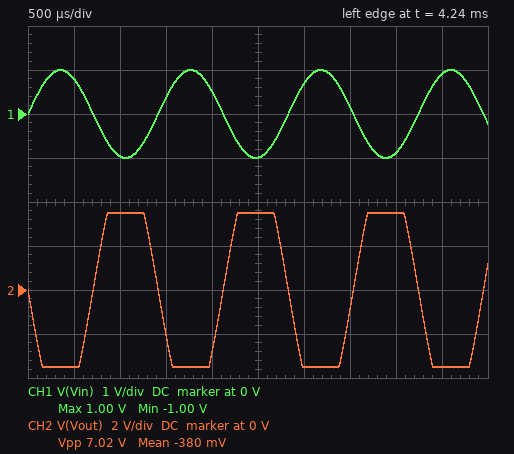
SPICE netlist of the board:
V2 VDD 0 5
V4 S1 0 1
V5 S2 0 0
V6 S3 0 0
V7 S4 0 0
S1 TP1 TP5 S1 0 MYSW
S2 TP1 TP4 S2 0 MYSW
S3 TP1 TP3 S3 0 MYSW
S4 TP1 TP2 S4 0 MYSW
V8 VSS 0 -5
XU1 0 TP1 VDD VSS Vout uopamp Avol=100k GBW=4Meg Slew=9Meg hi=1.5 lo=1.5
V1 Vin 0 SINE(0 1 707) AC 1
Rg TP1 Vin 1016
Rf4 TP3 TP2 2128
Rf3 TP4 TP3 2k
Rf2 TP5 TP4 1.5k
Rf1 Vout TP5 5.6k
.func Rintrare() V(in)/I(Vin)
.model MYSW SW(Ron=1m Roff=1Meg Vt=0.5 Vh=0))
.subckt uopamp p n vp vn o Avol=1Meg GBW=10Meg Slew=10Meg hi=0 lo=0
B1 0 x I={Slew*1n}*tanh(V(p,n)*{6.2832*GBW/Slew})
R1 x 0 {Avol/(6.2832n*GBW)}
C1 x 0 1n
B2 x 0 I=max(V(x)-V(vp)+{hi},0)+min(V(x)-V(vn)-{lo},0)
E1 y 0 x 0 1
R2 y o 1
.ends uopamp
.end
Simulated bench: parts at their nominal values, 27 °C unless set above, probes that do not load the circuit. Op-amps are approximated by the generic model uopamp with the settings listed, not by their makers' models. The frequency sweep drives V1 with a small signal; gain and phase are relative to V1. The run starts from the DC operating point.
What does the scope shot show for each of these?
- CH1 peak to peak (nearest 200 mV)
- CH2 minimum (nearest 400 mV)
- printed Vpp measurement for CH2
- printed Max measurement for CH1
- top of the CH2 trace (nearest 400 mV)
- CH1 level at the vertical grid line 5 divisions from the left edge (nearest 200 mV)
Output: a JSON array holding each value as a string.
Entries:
["2.0 V", "-3.6 V", "7.02 V", "1.00 V", "3.6 V", "-1.0 V"]
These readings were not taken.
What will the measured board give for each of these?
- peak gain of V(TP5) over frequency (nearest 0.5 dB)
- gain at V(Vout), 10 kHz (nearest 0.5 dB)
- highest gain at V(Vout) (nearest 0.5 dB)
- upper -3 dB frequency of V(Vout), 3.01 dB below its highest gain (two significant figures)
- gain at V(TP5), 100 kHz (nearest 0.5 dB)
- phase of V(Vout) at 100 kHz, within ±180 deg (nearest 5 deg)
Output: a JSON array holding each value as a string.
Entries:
["48.0 dB", "46.5 dB", "48.0 dB", "16 kHz", "31.5 dB", "100 deg"]
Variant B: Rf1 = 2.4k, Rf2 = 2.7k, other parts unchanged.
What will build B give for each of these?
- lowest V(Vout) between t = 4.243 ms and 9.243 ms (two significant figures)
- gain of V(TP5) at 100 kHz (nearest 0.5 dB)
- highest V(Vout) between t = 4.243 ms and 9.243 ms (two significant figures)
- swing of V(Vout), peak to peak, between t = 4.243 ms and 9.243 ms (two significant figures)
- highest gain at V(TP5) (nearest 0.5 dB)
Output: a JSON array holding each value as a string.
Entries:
["-2.4 V", "32.0 dB", "2.4 V", "4.7 V", "48.0 dB"]
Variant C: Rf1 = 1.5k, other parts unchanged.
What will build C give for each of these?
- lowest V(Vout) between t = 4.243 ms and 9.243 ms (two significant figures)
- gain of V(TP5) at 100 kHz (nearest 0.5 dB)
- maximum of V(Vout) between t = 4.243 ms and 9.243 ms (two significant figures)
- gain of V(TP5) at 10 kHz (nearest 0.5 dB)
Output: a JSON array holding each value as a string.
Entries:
["-1.5 V", "32.0 dB", "1.5 V", "46.5 dB"]
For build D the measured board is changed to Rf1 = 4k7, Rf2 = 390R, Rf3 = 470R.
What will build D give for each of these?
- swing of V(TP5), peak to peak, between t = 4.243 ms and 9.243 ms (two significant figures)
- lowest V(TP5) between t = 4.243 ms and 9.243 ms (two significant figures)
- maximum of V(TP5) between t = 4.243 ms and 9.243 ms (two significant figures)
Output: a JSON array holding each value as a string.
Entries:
["400 mV", "-200 mV", "200 mV"]
